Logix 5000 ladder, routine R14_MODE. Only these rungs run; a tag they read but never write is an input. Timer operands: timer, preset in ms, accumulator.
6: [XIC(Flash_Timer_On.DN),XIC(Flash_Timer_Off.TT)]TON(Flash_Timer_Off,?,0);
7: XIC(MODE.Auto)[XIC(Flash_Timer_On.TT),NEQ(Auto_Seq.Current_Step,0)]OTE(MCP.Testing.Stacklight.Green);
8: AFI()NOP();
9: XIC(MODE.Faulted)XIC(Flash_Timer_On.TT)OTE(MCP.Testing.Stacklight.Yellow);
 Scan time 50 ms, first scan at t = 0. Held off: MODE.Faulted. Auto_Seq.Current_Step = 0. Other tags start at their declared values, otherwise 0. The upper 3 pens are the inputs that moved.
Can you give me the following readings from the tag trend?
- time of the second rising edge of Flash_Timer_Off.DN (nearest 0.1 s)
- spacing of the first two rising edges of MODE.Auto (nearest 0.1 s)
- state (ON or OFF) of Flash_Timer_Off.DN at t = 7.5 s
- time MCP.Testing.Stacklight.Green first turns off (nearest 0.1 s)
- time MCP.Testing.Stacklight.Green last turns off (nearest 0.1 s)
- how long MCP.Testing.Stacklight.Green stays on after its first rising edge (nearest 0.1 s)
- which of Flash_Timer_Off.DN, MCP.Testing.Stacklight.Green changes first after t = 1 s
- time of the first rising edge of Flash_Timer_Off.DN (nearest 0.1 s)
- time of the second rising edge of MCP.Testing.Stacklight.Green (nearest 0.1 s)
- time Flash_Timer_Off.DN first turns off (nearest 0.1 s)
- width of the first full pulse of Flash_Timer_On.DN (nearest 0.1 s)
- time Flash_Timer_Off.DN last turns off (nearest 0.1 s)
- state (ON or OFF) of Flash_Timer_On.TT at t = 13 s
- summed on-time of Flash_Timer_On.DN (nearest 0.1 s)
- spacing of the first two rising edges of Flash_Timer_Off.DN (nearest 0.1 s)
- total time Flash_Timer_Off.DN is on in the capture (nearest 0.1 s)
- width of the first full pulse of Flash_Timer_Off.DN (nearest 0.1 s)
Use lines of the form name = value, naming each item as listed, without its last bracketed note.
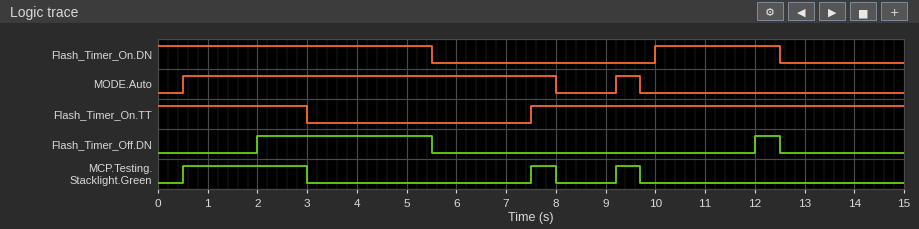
time of the second rising edge of Flash_Timer_Off.DN = 12.0 s
spacing of the first two rising edges of MODE.Auto = 8.7 s
state (ON or OFF) of Flash_Timer_Off.DN at t = 7.5 s = OFF
time MCP.Testing.Stacklight.Green first turns off = 3.0 s
time MCP.Testing.Stacklight.Green last turns off = 9.7 s
how long MCP.Testing.Stacklight.Green stays on after its first rising edge = 2.5 s
which of Flash_Timer_Off.DN, MCP.Testing.Stacklight.Green changes first after t = 1 s = Flash_Timer_Off.DN
time of the first rising edge of Flash_Timer_Off.DN = 2.0 s
time of the second rising edge of MCP.Testing.Stacklight.Green = 7.5 s
time Flash_Timer_Off.DN first turns off = 5.5 s
width of the first full pulse of Flash_Timer_On.DN = 2.5 s
time Flash_Timer_Off.DN last turns off = 12.5 s
state (ON or OFF) of Flash_Timer_On.TT at t = 13 s = ON
summed on-time of Flash_Timer_On.DN = 8.0 s
spacing of the first two rising edges of Flash_Timer_Off.DN = 10.0 s
total time Flash_Timer_Off.DN is on in the capture = 4.0 s
width of the first full pulse of Flash_Timer_Off.DN = 3.5 s
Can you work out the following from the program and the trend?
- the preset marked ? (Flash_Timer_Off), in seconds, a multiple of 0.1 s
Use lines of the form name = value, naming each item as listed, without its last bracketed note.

the preset marked ? (Flash_Timer_Off), in seconds, a multiple of 0.1 s = 2.0 s
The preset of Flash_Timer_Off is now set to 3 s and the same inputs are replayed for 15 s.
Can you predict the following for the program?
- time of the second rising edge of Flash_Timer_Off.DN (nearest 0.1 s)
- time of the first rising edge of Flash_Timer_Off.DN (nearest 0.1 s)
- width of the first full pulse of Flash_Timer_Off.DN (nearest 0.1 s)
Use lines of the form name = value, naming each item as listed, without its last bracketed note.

time of the second rising edge of Flash_Timer_Off.DN = 13.0 s
time of the first rising edge of Flash_Timer_Off.DN = 3.0 s
width of the first full pulse of Flash_Timer_Off.DN = 2.5 s
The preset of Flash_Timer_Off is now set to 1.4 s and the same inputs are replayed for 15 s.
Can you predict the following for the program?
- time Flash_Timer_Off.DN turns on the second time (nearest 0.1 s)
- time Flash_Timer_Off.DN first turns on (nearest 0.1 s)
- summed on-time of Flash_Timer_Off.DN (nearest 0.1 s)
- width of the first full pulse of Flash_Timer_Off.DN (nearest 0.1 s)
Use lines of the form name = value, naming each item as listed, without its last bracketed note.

time Flash_Timer_Off.DN turns on the second time = 11.4 s
time Flash_Timer_Off.DN first turns on = 1.4 s
summed on-time of Flash_Timer_Off.DN = 5.2 s
width of the first full pulse of Flash_Timer_Off.DN = 4.1 s
